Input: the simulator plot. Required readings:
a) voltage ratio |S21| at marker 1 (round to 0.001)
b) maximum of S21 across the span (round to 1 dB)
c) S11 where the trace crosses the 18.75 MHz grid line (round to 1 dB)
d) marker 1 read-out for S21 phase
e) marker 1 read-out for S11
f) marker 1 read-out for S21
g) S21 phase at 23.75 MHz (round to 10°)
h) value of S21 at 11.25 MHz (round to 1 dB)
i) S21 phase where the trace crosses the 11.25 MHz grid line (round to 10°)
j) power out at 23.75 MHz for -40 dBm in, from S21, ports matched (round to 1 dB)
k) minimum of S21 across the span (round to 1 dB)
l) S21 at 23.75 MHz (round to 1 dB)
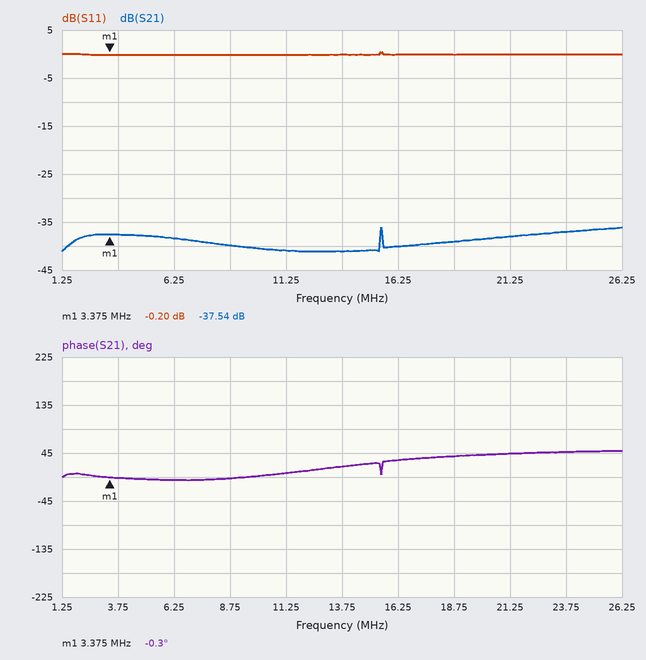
0.013
-36 dB
0 dB
-0.3°
-0.20 dB
-37.54 dB
50°
-41 dB
10°
-77 dBm
-41 dB
-37 dB
